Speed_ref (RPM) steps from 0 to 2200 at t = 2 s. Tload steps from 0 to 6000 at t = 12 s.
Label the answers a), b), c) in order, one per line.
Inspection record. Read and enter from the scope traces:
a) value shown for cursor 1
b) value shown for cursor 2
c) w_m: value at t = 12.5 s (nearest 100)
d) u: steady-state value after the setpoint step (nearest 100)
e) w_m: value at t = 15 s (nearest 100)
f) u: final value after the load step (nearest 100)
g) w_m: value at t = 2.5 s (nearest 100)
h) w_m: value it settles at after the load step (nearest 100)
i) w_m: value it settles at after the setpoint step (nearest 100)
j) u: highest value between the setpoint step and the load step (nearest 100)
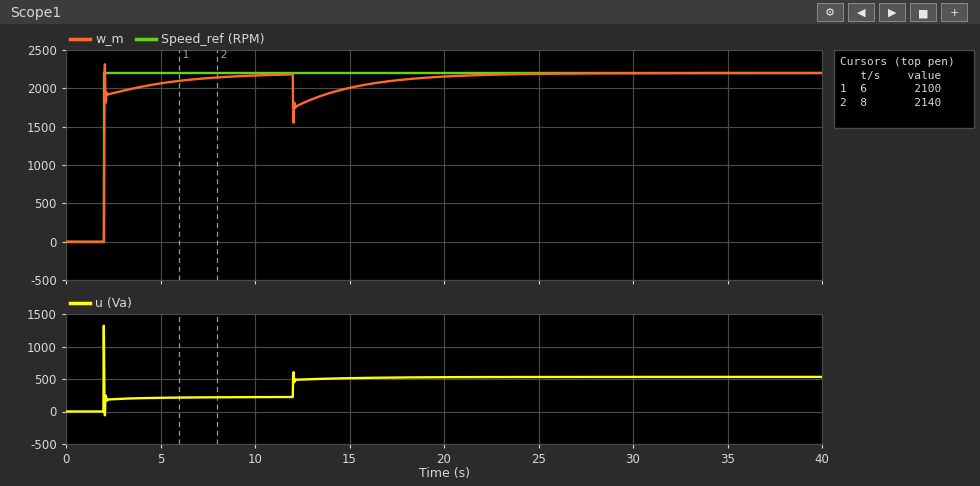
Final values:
a) 2100
b) 2140
c) 1800
d) 200
e) 2000
f) 500
g) 1900
h) 2200
i) 2200
j) 1300
